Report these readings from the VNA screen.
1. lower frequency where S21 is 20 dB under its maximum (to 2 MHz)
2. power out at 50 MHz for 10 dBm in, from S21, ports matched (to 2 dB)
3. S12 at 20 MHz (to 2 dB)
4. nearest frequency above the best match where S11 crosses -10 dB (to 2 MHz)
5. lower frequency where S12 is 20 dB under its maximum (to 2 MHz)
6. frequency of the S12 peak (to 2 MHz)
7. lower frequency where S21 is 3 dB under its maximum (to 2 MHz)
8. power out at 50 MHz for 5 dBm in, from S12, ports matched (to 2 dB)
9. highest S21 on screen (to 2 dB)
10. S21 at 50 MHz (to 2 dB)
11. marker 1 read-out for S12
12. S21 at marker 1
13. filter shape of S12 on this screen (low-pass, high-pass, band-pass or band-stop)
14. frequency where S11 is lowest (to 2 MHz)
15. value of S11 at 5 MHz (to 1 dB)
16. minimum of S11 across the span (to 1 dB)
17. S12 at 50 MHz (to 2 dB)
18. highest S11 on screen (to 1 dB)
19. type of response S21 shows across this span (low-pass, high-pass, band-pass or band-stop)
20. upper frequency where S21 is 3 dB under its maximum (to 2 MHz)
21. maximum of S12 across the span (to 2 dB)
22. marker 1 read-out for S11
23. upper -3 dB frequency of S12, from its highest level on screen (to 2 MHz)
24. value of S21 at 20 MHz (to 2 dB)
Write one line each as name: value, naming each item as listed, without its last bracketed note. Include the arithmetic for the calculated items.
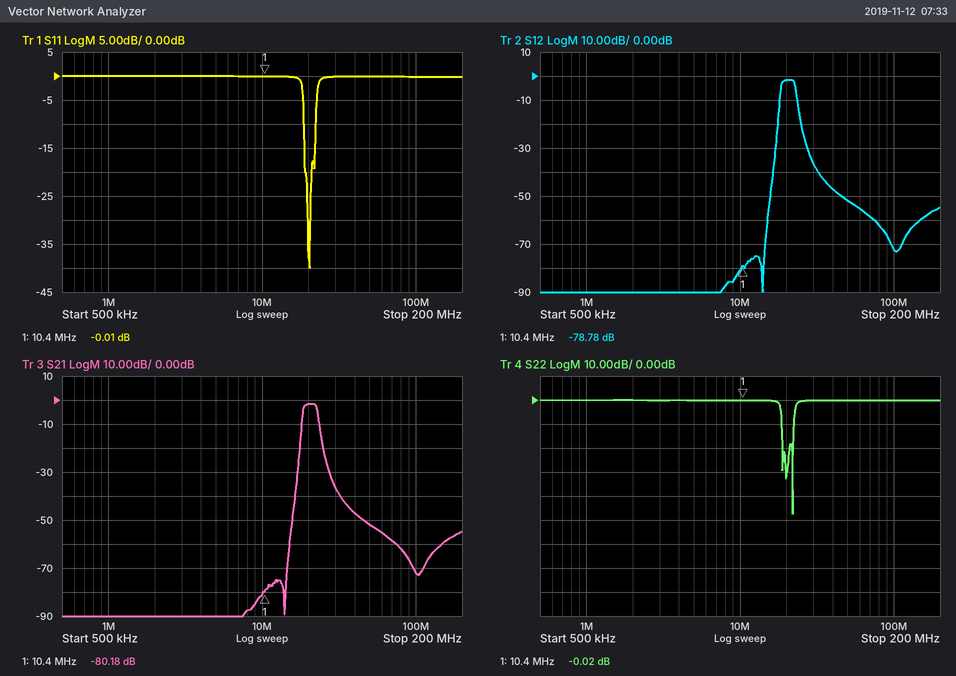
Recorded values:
lower frequency where S21 is 20 dB under its maximum: 18 MHz
power out at 50 MHz for 10 dBm in, from S21, ports matched: 10 dBm + (-52 dB) = -42 dBm
S12 at 20 MHz: -2 dB
nearest frequency above the best match where S11 crosses -10 dB: 22 MHz
lower frequency where S12 is 20 dB under its maximum: 18 MHz
frequency of the S12 peak: 20 MHz
lower frequency where S21 is 3 dB under its maximum: 18 MHz
power out at 50 MHz for 5 dBm in, from S12, ports matched: 5 dBm + (-52 dB) = -46 dBm
highest S21 on screen: -2 dB
S21 at 50 MHz: -52 dB
marker 1 read-out for S12: -78.78 dB
S21 at marker 1: -80.18 dB
filter shape of S12 on this screen: band-pass
frequency where S11 is lowest: 20 MHz
value of S11 at 5 MHz: 0 dB
minimum of S11 across the span: -40 dB
S12 at 50 MHz: -52 dB
highest S11 on screen: 0 dB
type of response S21 shows across this span: band-pass
upper frequency where S21 is 3 dB under its maximum: 22 MHz
maximum of S12 across the span: -2 dB
marker 1 read-out for S11: -0.01 dB
upper -3 dB frequency of S12, from its highest level on screen: 22 MHz
value of S21 at 20 MHz: -2 dB
